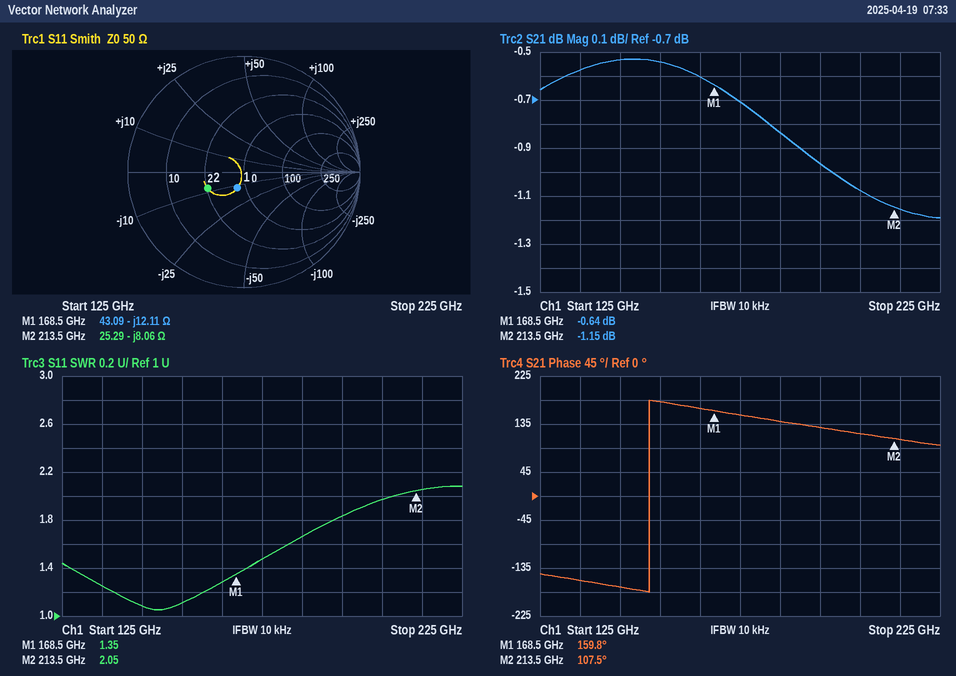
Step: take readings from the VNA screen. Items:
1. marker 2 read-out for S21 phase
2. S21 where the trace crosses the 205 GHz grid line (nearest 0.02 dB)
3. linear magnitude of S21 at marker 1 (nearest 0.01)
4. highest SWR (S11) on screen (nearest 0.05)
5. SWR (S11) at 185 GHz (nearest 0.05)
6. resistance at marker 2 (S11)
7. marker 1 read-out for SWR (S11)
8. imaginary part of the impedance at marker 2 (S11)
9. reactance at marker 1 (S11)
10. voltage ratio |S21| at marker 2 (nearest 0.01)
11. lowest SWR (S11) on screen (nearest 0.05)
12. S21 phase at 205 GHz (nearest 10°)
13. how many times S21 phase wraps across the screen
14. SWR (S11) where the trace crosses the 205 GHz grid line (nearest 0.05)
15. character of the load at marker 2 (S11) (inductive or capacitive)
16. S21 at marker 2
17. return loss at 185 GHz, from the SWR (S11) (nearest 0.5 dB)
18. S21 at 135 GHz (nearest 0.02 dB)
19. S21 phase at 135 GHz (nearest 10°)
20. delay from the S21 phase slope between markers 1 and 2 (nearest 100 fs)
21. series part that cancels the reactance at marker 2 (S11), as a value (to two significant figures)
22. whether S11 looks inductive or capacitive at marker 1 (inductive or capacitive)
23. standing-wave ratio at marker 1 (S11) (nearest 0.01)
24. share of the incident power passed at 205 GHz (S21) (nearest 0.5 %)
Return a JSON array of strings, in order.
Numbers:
["107.5°", "-1.08 dB", "0.93", "2.10", "1.65", "25.29 Ω", "1.35", "-8.06 Ω", "-12.11 Ω", "0.88", "1.05", "120°", "1", "1.95", "capacitive", "-1.15 dB", "12.0 dB", "-0.58 dB", "-160°", "3.2 ps", "6.0 pH", "capacitive", "1.35", "78.0 %"]
